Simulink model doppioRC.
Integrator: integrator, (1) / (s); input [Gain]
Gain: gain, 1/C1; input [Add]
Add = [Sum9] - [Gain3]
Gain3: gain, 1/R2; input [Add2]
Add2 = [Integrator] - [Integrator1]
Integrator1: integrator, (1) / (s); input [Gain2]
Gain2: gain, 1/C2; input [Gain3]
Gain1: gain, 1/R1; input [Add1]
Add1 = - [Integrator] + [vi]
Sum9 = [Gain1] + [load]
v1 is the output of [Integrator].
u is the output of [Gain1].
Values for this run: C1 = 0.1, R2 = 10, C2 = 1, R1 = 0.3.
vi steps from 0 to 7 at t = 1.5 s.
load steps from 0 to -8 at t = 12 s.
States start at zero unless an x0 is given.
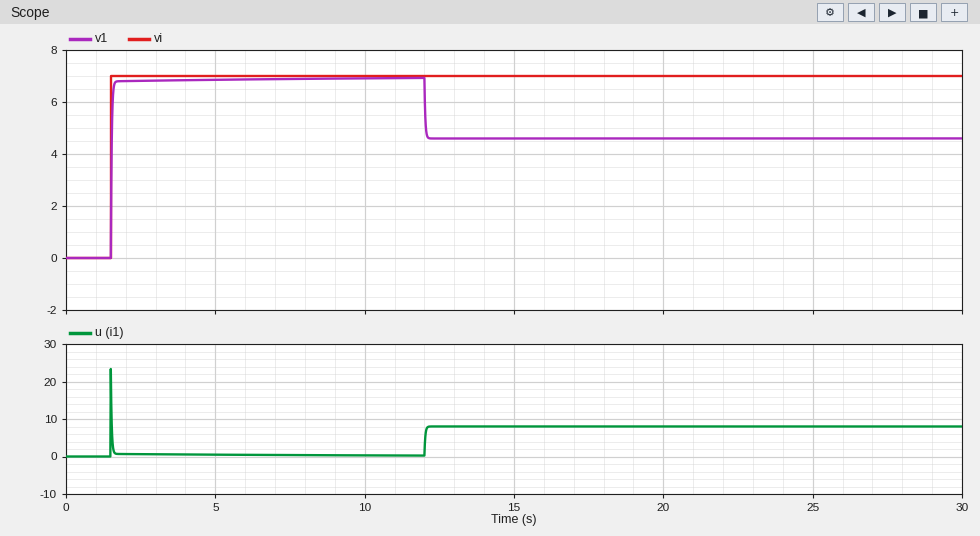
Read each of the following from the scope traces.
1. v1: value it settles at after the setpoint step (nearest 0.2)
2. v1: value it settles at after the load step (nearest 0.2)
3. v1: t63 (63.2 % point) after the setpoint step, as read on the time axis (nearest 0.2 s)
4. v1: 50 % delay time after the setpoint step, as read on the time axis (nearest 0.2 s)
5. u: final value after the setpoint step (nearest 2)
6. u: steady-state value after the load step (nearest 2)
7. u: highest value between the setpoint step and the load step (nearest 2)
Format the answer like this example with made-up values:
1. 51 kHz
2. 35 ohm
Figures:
1. 7.0
2. 4.6
3. 1.6 s
4. 1.6 s
5. 0
6. 8
7. 24
